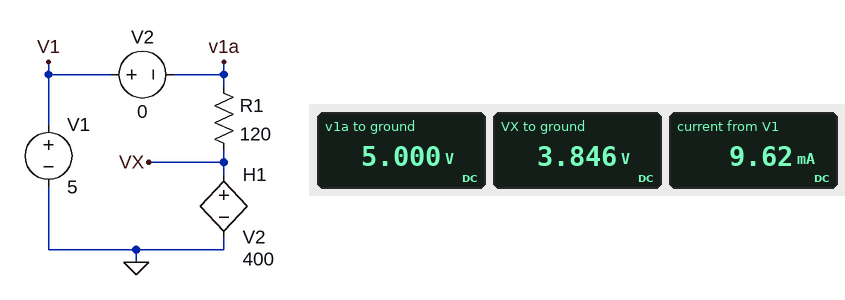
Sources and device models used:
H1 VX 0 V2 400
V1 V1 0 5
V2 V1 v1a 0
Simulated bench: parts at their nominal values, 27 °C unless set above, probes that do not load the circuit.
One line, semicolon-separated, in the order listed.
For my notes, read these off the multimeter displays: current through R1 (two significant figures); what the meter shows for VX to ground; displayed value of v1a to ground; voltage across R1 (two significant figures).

9.6 mA; 3.846 V; 5.000 V; 1.2 V
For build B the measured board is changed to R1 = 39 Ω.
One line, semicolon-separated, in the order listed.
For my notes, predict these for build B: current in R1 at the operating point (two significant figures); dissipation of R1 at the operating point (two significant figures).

11 mA; 5.1 mW
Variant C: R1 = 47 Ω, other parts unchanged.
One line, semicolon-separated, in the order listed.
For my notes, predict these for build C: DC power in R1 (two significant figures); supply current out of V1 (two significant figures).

5.9 mW; 11 mA
